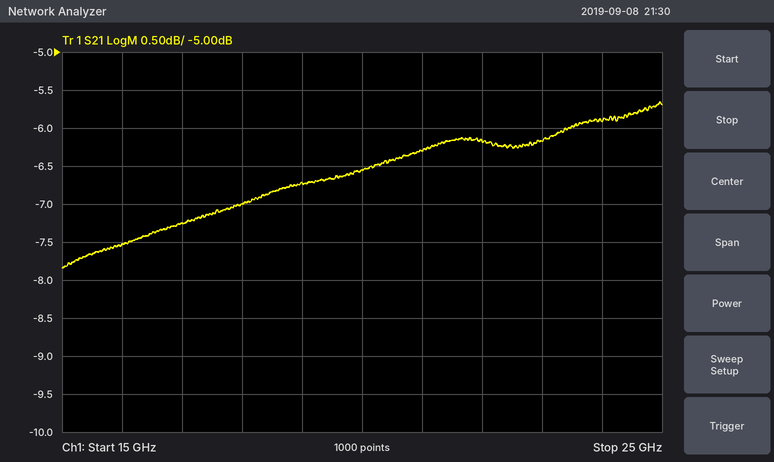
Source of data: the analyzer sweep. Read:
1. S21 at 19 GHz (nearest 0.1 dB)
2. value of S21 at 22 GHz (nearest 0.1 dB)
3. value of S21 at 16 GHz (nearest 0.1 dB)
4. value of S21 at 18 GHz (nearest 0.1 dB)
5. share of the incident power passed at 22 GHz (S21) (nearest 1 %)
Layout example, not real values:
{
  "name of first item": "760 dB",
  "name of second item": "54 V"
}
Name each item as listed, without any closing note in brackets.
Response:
{
  "S21 at 19 GHz": "-6.7 dB",
  "value of S21 at 22 GHz": "-6.2 dB",
  "value of S21 at 16 GHz": "-7.5 dB",
  "value of S21 at 18 GHz": "-7.0 dB",
  "share of the incident power passed at 22 GHz (S21)": "24 %"
}
